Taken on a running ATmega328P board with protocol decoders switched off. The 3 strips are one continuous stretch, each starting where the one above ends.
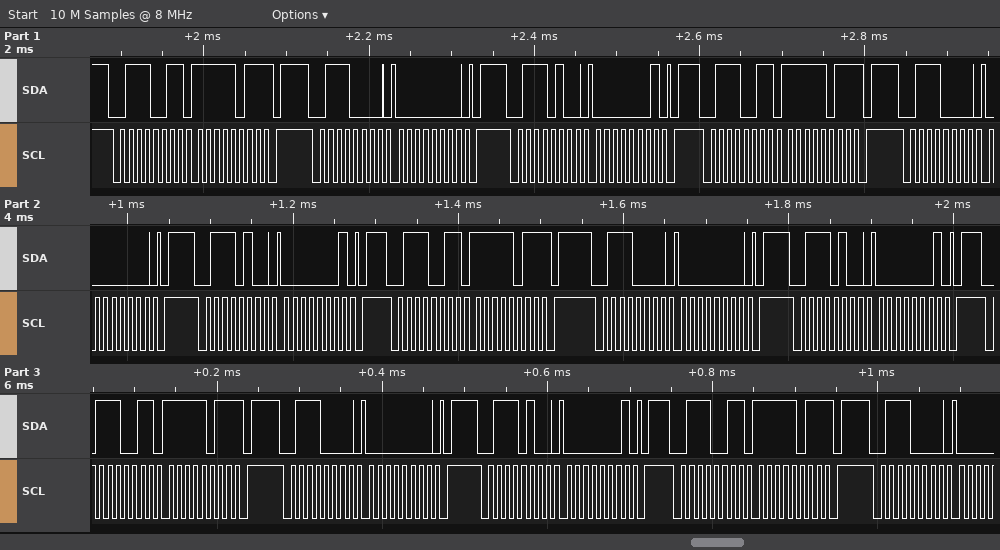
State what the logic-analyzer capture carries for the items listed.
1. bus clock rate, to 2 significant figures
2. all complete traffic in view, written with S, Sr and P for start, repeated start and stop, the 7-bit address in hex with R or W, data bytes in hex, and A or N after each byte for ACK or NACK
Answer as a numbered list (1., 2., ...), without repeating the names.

1. 100 kHz
2. S 39R A FB N P S 38W A 00 A P S 3AW A 01 A P S 39R A FB N P S 38W A 00 A P S 3AW A 01 A P S 39R A FB N P S 38W A 00 A P S 3AW A 01 A P S 39R A FB N P S 38W A 00 A P S 3AW A 01 A P S 39R A FB N P S 38W A
